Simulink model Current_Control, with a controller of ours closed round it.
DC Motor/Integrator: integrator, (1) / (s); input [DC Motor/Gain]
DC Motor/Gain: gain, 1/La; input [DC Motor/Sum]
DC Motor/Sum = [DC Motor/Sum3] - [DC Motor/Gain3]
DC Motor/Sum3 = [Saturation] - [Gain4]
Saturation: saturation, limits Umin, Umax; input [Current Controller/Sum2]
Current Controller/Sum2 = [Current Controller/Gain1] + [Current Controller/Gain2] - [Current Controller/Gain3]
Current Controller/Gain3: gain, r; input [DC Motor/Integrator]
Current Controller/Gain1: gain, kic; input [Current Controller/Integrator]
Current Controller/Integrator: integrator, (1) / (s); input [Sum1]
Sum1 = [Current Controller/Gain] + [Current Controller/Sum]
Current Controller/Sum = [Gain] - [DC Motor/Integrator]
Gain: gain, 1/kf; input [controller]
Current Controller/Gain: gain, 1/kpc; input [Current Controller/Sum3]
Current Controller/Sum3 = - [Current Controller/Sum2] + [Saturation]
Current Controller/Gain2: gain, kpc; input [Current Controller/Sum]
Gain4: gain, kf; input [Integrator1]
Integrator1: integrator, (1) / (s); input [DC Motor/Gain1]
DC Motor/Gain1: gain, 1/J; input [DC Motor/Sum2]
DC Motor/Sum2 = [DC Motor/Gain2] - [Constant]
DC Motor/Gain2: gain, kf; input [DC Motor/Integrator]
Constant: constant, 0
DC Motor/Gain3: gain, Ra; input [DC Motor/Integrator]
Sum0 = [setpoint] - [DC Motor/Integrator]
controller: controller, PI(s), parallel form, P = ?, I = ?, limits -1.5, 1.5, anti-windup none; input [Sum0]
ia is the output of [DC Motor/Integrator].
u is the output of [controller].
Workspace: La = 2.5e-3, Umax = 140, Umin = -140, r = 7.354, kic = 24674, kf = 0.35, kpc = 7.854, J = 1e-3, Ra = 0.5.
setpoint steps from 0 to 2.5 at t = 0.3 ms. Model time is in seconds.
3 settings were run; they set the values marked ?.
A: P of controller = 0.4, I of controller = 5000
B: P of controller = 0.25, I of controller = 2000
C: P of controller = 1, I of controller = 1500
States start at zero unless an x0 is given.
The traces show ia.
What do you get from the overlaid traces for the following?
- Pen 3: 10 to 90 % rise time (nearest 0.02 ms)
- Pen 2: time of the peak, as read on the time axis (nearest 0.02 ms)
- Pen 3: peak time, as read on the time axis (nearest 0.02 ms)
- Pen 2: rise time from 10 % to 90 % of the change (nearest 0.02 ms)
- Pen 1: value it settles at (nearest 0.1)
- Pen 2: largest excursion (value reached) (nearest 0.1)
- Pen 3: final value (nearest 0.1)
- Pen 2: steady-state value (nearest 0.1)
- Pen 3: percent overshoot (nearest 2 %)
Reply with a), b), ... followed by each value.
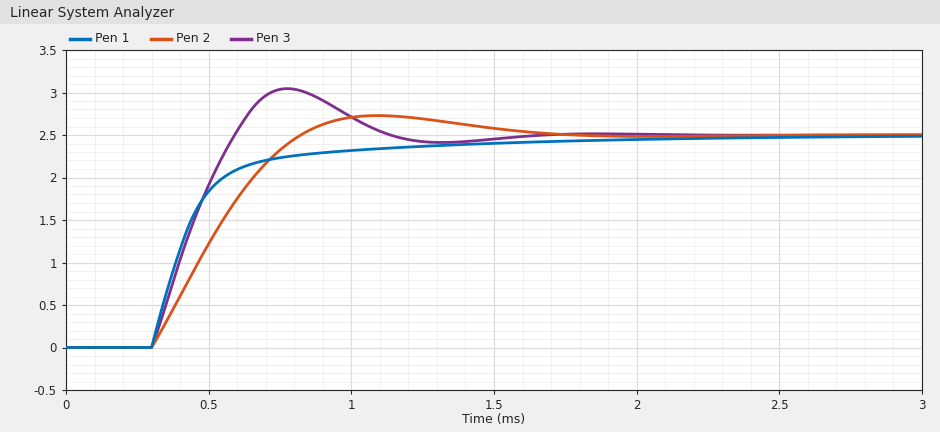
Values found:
a) 0.22 ms
b) 1.10 ms
c) 0.78 ms
d) 0.38 ms
e) 2.5
f) 2.7
g) 2.5
h) 2.5
i) 22 %
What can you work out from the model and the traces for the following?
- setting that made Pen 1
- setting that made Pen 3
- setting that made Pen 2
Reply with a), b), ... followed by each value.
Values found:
a) C
b) A
c) B
